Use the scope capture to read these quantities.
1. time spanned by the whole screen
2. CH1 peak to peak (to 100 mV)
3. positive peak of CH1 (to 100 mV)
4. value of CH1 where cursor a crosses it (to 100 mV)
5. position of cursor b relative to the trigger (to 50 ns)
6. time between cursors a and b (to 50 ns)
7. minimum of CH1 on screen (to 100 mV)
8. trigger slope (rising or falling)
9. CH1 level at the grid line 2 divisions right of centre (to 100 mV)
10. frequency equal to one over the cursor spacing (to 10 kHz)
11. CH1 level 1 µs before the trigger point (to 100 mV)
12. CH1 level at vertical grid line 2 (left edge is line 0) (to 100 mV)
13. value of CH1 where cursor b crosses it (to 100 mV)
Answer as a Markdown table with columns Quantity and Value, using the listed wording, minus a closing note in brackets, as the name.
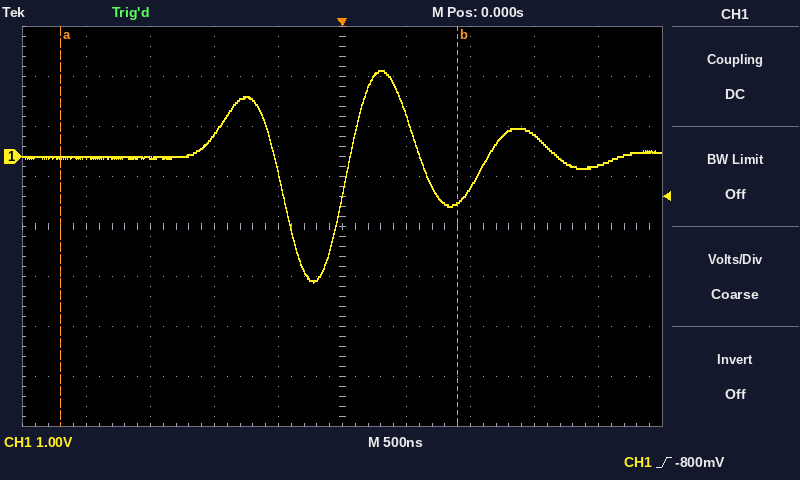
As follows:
| Quantity | Value |
|---|---|
| time spanned by the whole screen | 5 µs |
| CH1 peak to peak | 4.2 V |
| positive peak of CH1 | 1.7 V |
| value of CH1 where cursor a crosses it | 0.0 V |
| position of cursor b relative to the trigger | +900 ns |
| time between cursors a and b | 3.10 µs |
| minimum of CH1 on screen | -2.5 V |
| trigger slope | rising |
| CH1 level at the grid line 2 divisions right of centre | -600 mV |
| frequency equal to one over the cursor spacing | 320 kHz |
| CH1 level 1 µs before the trigger point | 400 mV |
| CH1 level at vertical grid line 2 (left edge is line 0) | 0.0 V |
| value of CH1 where cursor b crosses it | -900 mV |
